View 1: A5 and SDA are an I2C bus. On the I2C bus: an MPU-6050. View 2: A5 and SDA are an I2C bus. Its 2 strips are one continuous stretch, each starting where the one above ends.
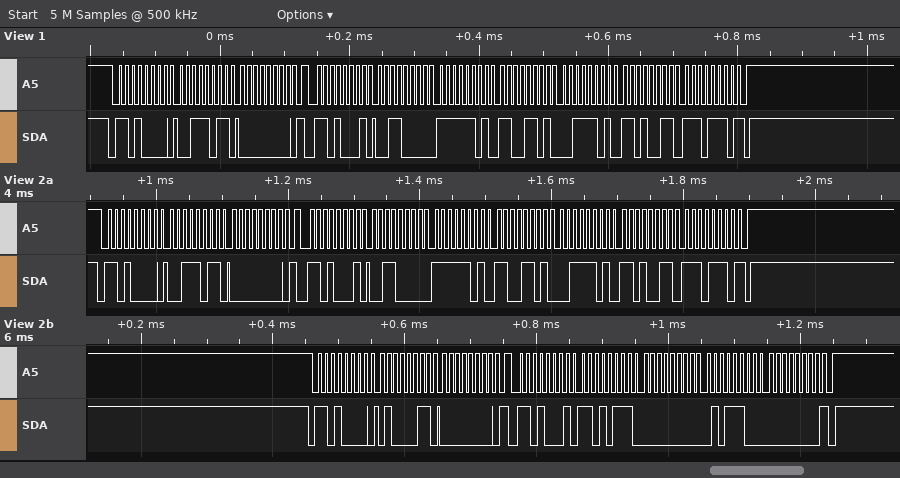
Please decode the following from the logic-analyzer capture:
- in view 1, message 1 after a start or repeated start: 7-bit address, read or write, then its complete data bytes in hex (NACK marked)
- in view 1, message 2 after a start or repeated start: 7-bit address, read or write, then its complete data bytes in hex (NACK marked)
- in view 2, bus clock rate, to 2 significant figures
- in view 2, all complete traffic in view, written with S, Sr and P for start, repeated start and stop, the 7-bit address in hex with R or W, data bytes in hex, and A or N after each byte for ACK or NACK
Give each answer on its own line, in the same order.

0x68 write: 3B 00
0x68 read: 30 FD CD 3D D3 EE NACK
100 kHz
S 68W A 3B A 00 A Sr 68R A 30 A FD A CD A 3D A D3 A EE N P S 68W A 43 A 00 A Sr 68R A D7 A 00 A 5C A 00 N P
